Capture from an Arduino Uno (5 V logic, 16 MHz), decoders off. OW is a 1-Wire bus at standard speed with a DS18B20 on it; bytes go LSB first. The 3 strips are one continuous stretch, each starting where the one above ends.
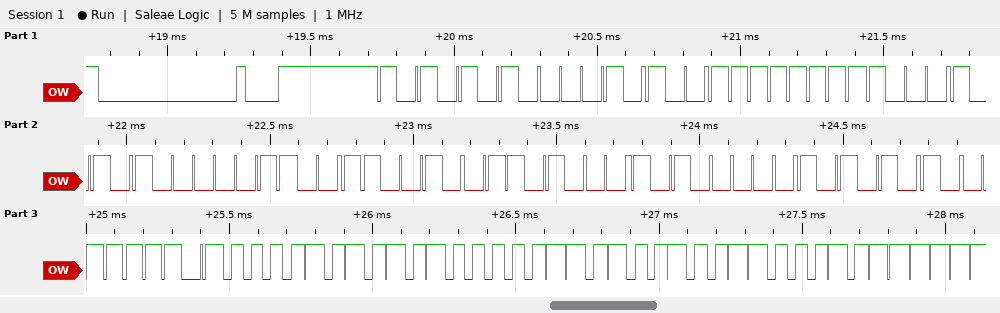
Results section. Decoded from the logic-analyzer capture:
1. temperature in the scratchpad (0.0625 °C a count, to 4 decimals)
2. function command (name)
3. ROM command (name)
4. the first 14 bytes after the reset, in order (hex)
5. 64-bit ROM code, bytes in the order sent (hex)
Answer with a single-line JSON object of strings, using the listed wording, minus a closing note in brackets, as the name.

{"temperature in the scratchpad": "85.0000 °C", "function command": "Read Scratchpad", "ROM command": "Match ROM", "the first 14 bytes after the reset, in order": "55 28 FF 51 C1 4C 16 05 55 BE 50 05 4B 46", "64-bit ROM code, bytes in the order sent": "28 FF 51 C1 4C 16 05 55"}
